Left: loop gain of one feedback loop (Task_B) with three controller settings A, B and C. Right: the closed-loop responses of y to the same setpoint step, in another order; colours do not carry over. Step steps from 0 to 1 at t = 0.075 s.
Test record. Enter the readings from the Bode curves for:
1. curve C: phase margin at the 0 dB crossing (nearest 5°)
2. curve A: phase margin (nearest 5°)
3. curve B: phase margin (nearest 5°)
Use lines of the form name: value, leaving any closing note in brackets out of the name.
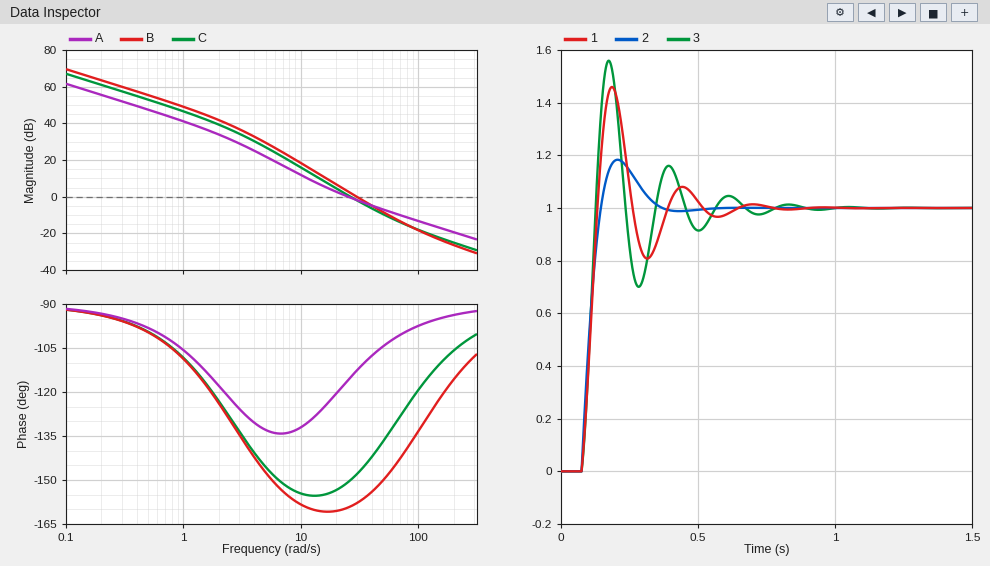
curve C: phase margin at the 0 dB crossing: 30°
curve A: phase margin: 65°
curve B: phase margin: 20°
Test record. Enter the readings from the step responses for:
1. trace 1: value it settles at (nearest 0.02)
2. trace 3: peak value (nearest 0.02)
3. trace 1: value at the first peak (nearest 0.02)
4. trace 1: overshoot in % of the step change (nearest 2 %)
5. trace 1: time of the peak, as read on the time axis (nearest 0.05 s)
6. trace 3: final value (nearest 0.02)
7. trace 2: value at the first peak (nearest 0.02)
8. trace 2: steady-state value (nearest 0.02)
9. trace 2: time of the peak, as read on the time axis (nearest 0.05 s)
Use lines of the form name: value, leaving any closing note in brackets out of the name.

trace 1: value it settles at: 1.00
trace 3: peak value: 1.56
trace 1: value at the first peak: 1.46
trace 1: overshoot in % of the step change: 46 %
trace 1: time of the peak, as read on the time axis: 0.20 s
trace 3: final value: 1.00
trace 2: value at the first peak: 1.18
trace 2: steady-state value: 1.00
trace 2: time of the peak, as read on the time axis: 0.20 s
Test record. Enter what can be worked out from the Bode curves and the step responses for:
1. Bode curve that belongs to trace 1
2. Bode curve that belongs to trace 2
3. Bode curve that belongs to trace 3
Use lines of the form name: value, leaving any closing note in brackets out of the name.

Bode curve that belongs to trace 1: C
Bode curve that belongs to trace 2: A
Bode curve that belongs to trace 3: B
